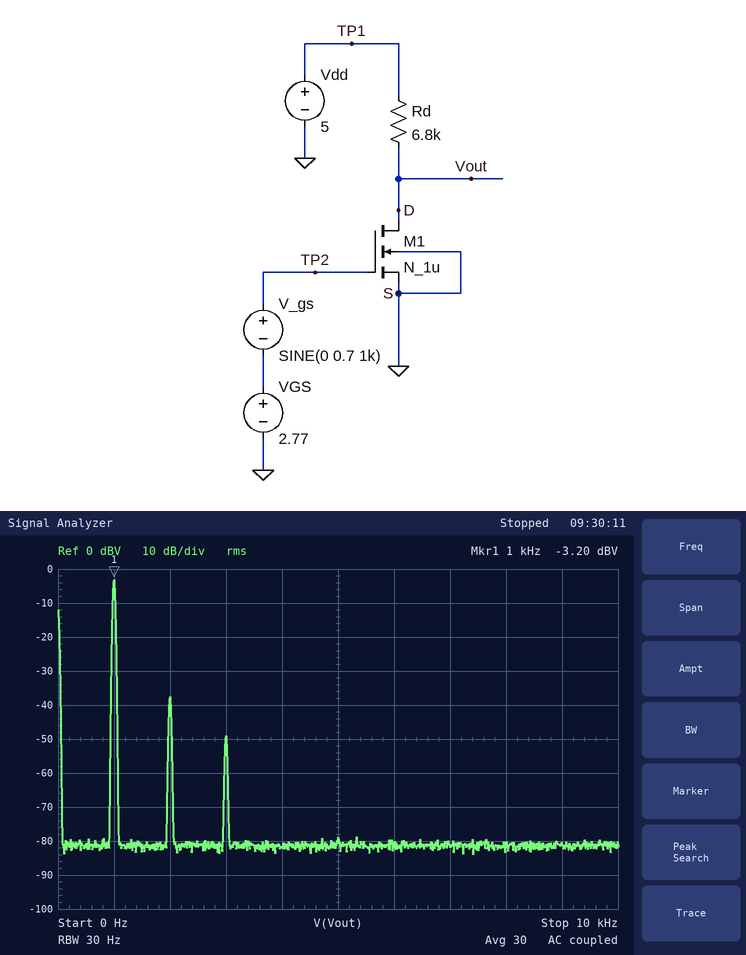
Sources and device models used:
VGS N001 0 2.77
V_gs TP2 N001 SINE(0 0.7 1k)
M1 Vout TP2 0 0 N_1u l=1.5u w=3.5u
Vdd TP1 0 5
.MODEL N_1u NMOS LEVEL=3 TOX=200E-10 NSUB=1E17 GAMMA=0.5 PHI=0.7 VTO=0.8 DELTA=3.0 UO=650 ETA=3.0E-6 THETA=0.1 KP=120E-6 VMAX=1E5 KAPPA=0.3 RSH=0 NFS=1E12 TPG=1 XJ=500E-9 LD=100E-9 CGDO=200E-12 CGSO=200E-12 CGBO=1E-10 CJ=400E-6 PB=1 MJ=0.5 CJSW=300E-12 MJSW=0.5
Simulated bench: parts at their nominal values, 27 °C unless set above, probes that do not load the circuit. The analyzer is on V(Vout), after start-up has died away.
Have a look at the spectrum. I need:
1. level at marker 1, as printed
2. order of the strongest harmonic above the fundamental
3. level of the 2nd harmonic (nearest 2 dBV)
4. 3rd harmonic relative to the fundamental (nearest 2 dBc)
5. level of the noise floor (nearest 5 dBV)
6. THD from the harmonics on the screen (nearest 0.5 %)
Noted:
-3.20 dBV
2
-38 dBV
-46 dBc
-80 dBV
2.0 %
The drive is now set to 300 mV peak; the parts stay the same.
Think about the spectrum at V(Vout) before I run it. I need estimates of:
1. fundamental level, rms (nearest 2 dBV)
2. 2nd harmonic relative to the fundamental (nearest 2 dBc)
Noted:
-10 dBV
-42 dBc
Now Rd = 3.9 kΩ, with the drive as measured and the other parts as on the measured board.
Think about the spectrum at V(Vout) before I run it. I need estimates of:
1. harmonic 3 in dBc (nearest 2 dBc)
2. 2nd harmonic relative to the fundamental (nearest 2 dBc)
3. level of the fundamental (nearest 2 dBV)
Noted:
-48 dBc
-32 dBc
-8 dBV
